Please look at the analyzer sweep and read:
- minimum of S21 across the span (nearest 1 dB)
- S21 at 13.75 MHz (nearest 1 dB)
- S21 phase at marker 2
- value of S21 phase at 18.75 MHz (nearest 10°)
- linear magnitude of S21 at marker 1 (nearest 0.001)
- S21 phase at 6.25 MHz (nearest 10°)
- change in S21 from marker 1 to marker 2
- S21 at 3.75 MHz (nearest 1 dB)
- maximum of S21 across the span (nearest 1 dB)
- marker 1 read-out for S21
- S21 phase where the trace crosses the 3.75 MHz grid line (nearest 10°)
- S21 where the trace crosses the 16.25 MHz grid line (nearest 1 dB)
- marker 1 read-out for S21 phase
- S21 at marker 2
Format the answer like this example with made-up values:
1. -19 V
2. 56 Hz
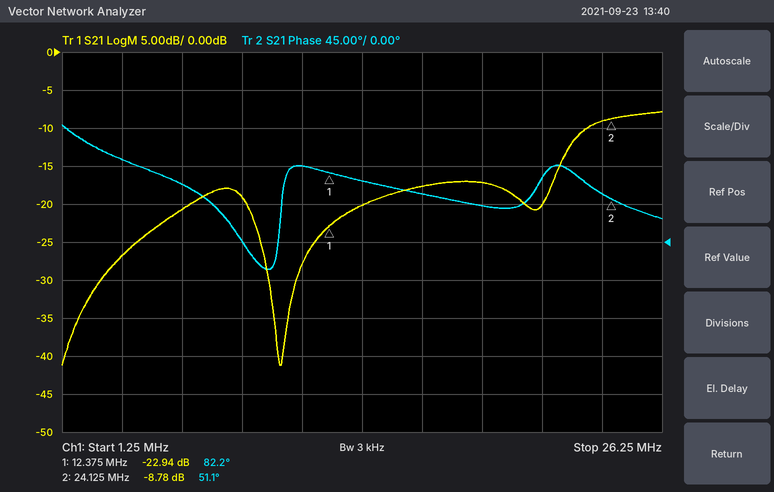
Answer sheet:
1. -41 dB
2. -20 dB
3. 51.1°
4. 40°
5. 0.071
6. 70°
7. 14.16 dB
8. -27 dB
9. -8 dB
10. -22.94 dB
11. 100°
12. -18 dB
13. 82.2°
14. -8.78 dB
